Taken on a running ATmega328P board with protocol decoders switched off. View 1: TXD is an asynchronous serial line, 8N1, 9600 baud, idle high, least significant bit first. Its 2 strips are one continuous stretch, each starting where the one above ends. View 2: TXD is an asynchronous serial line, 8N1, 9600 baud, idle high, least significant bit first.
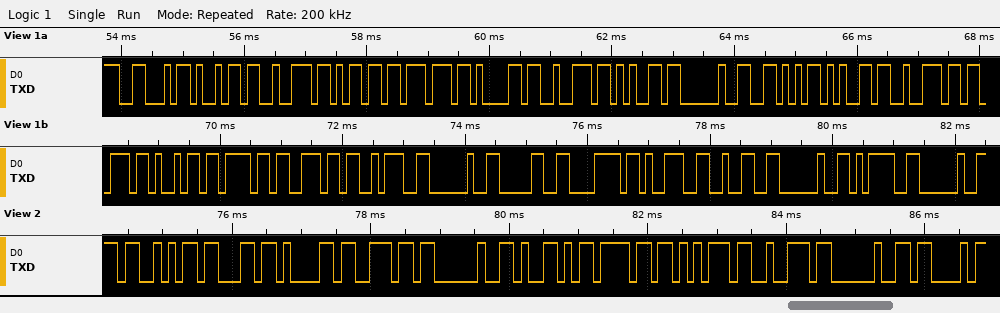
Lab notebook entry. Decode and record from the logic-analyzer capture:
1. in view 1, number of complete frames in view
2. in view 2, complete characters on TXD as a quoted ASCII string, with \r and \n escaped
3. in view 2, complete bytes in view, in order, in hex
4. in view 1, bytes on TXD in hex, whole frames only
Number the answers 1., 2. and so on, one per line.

1. 25
2. "Scan Your C"
3. 53 63 61 6E 20 59 6F 75 72 20 43
4. 46 69 72 6D 77 61 72 65 20 56 65 72 73 69 6F 6E 3A 20 30 78 39 32 20 3D 20
